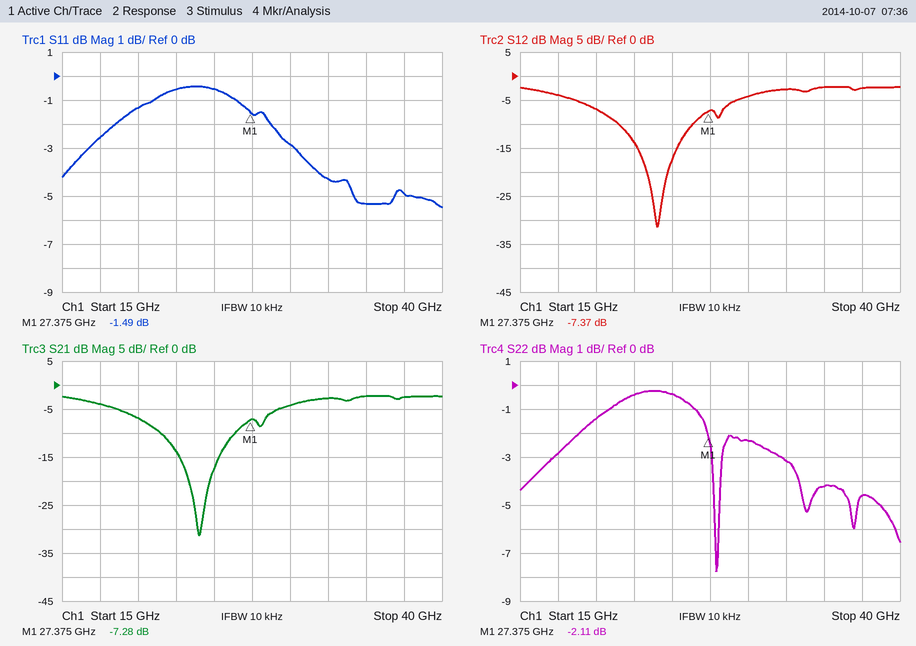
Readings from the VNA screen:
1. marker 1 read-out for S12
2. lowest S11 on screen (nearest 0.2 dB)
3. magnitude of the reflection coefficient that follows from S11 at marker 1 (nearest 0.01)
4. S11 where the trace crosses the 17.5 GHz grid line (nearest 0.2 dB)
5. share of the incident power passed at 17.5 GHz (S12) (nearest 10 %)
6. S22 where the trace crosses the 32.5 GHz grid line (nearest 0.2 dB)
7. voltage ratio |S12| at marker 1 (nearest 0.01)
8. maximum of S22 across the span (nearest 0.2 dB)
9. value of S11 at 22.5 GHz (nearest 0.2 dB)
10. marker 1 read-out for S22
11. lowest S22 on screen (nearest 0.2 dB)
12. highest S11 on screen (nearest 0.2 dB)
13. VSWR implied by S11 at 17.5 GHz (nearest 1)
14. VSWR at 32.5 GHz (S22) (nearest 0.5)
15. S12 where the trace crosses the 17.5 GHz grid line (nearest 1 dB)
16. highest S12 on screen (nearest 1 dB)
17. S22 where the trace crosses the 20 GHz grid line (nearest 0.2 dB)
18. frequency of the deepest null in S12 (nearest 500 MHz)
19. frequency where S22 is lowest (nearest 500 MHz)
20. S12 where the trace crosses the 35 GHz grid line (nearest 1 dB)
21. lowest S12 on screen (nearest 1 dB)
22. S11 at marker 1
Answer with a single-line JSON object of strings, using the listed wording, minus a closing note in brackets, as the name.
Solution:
{"marker 1 read-out for S12": "-7.37 dB", "lowest S11 on screen": "-5.4 dB", "magnitude of the reflection coefficient that follows from S11 at marker 1": "0.84", "S11 where the trace crosses the 17.5 GHz grid line": "-2.6 dB", "share of the incident power passed at 17.5 GHz (S12)": "40 %", "S22 where the trace crosses the 32.5 GHz grid line": "-3.2 dB", "voltage ratio |S12| at marker 1": "0.43", "maximum of S22 across the span": "-0.2 dB", "value of S11 at 22.5 GHz": "-0.6 dB", "marker 1 read-out for S22": "-2.11 dB", "lowest S22 on screen": "-7.8 dB", "highest S11 on screen": "-0.4 dB", "VSWR implied by S11 at 17.5 GHz": "7", "VSWR at 32.5 GHz (S22)": "5.5", "S12 where the trace crosses the 17.5 GHz grid line": "-4 dB", "highest S12 on screen": "-2 dB", "S22 where the trace crosses the 20 GHz grid line": "-1.4 dB", "frequency of the deepest null in S12": "24.0 GHz", "frequency where S22 is lowest": "28.0 GHz", "S12 where the trace crosses the 35 GHz grid line": "-2 dB", "lowest S12 on screen": "-31 dB", "S11 at marker 1": "-1.49 dB"}
